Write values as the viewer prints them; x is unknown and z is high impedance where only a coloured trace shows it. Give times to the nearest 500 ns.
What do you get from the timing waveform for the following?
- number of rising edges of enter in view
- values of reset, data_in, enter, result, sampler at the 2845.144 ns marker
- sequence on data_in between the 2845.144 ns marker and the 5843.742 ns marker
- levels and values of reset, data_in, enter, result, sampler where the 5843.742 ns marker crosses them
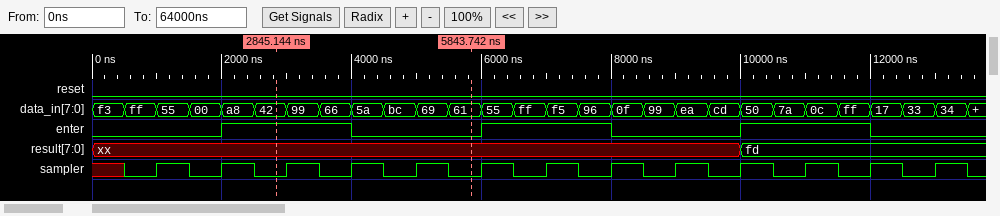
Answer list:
3
reset=0, data_in=42, enter=1, result=xx, sampler=0
42, 99, 66, 5a, bc, 69, 61
reset=0, data_in=61, enter=0, result=xx, sampler=0
